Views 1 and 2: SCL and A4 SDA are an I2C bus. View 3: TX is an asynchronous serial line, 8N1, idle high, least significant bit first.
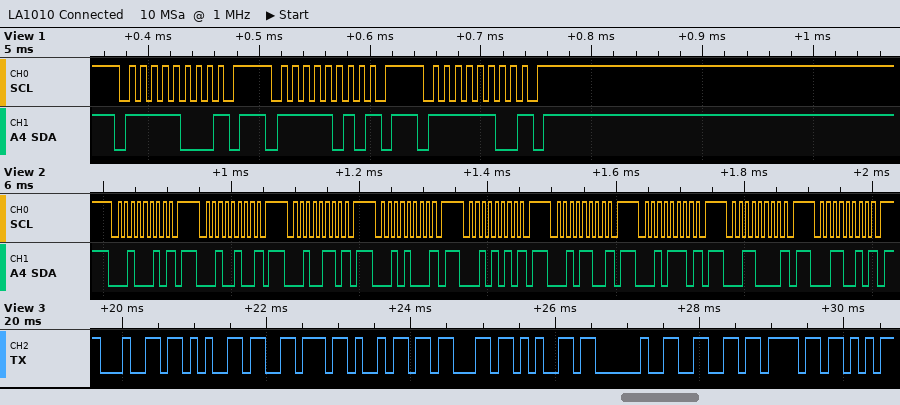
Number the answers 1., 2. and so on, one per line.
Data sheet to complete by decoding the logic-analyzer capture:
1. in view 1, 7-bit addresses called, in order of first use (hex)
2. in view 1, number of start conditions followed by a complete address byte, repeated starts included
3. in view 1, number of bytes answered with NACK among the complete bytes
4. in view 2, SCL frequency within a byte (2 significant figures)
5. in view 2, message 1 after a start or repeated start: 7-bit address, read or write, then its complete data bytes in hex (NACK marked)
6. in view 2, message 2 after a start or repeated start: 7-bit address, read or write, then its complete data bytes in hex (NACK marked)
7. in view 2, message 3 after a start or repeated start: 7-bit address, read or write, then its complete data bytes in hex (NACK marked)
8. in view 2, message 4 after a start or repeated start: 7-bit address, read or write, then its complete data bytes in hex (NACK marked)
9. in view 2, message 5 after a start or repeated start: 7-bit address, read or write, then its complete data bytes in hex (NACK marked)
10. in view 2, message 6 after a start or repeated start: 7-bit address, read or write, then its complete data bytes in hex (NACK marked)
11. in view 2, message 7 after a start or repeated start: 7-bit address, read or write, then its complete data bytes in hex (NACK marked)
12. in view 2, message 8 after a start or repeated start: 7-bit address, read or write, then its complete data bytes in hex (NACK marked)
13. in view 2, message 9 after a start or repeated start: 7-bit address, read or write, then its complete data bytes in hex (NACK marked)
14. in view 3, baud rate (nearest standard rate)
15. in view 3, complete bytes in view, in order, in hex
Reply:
1. 0x7C 0x7D 0x7E
2. 3
3. 3
4. 100 kHz
5. 0x11 write NACK
6. 0x12 write NACK
7. 0x13 write NACK
8. 0x14 write NACK
9. 0x15 write NACK
10. 0x16 write NACK
11. 0x17 write NACK
12. 0x18 write NACK
13. 0x19 write NACK
14. 9600 baud
15. 64 65 76 69 63 65 20 66 6F
